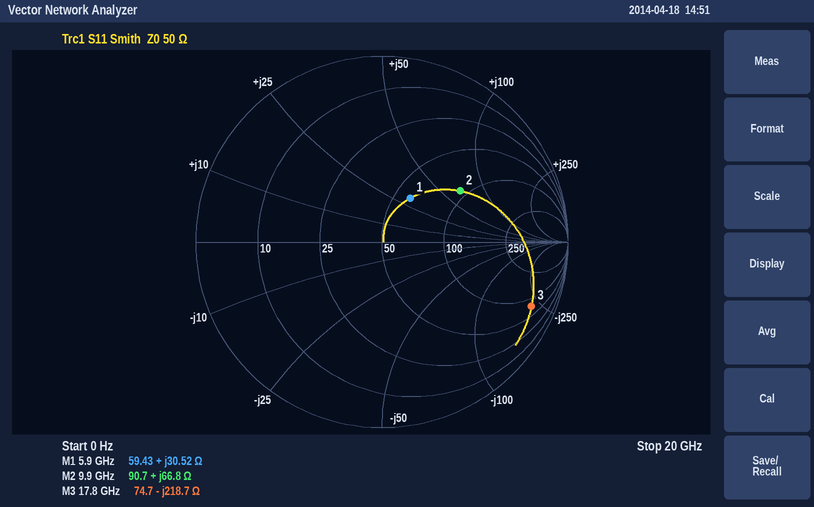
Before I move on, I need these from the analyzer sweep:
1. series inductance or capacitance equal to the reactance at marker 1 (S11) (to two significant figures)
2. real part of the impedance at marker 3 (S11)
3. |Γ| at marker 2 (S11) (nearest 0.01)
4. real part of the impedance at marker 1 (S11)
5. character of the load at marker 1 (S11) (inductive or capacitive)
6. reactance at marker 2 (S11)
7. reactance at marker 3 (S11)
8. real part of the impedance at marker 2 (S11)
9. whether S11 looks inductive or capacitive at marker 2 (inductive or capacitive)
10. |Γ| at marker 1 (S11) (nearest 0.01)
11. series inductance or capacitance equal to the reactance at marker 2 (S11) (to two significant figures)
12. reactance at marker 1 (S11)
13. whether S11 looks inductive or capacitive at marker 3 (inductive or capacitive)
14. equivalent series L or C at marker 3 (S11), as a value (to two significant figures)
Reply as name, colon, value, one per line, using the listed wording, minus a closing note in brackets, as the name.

series inductance or capacitance equal to the reactance at marker 1 (S11): 820 pH
real part of the impedance at marker 3: 74.7 Ω
|Γ| at marker 2 (S11): 0.50
real part of the impedance at marker 1: 59.43 Ω
character of the load at marker 1 (S11): inductive
reactance at marker 2: +66.8 Ω
reactance at marker 3: -218.7 Ω
real part of the impedance at marker 2: 90.7 Ω
whether S11 looks inductive or capacitive at marker 2: inductive
|Γ| at marker 1 (S11): 0.28
series inductance or capacitance equal to the reactance at marker 2 (S11): 1.1 nH
reactance at marker 1: +30.52 Ω
whether S11 looks inductive or capacitive at marker 3: capacitive
equivalent series L or C at marker 3 (S11), as a value: 41 fF
